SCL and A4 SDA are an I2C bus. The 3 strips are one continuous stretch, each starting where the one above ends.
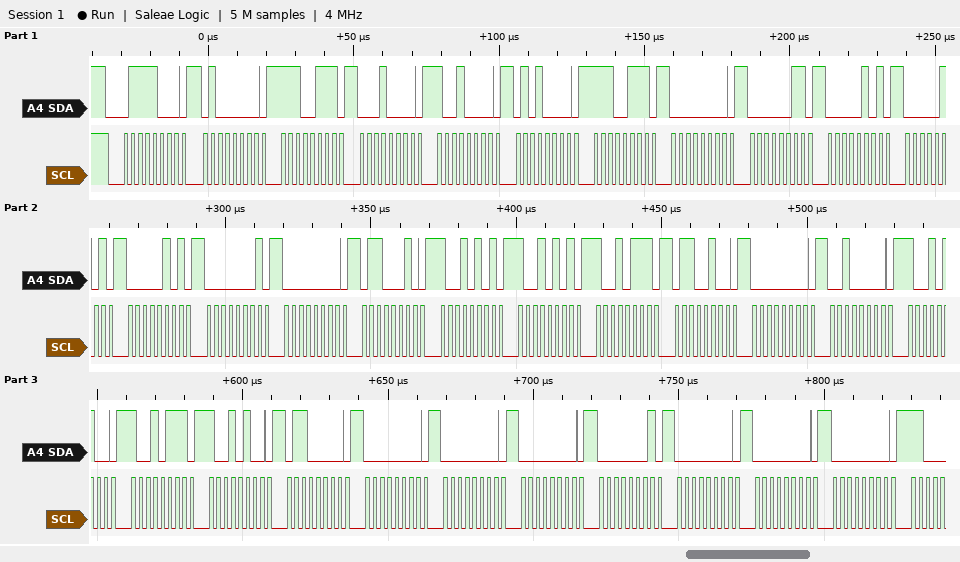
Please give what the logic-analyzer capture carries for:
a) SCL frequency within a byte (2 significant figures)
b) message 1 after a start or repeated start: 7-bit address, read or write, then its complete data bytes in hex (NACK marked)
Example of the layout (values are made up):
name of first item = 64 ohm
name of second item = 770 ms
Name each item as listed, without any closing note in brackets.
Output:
SCL frequency within a byte = 400 kHz
message 1 after a start or repeated start: 7-bit address, read or write, then its complete data bytes in hex = 0x3C write: 40 E7 10 90 50 E7 00 03 05 05 05 01 00 62 95 95 97 64 00 20 94 97 94 60 00 00 00 01 00 00 00
